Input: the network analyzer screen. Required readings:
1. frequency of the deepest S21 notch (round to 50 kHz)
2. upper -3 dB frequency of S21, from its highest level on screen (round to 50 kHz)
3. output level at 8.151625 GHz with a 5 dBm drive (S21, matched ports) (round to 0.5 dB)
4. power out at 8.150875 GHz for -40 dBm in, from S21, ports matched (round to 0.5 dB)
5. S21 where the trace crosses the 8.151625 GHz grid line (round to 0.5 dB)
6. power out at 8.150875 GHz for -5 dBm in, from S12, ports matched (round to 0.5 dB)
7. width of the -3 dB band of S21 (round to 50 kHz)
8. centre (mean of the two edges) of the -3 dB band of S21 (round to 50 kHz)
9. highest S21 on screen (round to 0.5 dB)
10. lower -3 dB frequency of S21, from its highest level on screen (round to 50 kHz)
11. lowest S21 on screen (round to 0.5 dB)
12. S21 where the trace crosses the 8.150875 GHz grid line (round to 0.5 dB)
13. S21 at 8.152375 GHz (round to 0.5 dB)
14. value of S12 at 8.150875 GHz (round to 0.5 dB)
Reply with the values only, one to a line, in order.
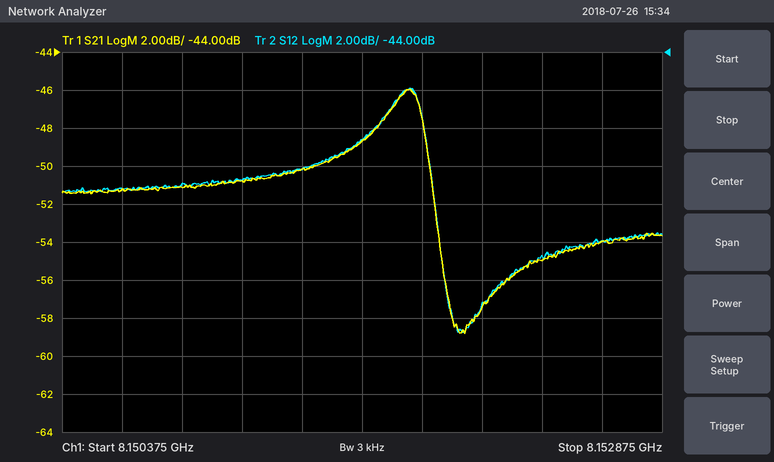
8.15205 GHz
8.15190 GHz
-43.5 dBm
-91.0 dBm
-48.5 dB
-56.0 dBm
300 kHz
8.15175 GHz
-46.0 dB
8.15160 GHz
-59.0 dB
-51.0 dB
-55.0 dB
-51.0 dB
